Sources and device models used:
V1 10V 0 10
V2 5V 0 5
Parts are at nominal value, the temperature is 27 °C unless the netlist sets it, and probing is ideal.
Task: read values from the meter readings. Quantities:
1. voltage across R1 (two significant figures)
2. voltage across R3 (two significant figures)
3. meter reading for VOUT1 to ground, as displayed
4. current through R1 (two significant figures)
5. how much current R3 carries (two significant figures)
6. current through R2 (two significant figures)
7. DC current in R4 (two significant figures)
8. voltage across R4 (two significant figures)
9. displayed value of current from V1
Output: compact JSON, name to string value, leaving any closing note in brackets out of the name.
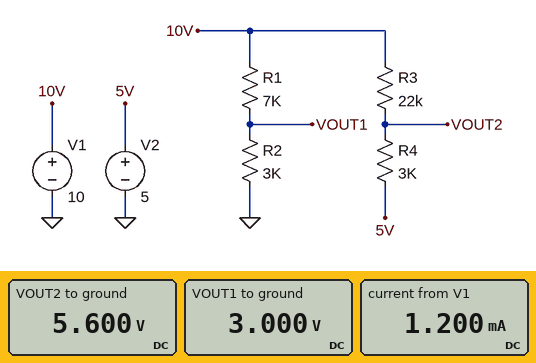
{"voltage across R1": "7.0 V", "voltage across R3": "4.4 V", "meter reading for VOUT1 to ground, as displayed": "3.000 V", "current through R1": "1.0 mA", "how much current R3 carries": "200 µA", "current through R2": "1.0 mA", "DC current in R4": "200 µA", "voltage across R4": "600 mV", "displayed value of current from V1": "1.200 mA"}
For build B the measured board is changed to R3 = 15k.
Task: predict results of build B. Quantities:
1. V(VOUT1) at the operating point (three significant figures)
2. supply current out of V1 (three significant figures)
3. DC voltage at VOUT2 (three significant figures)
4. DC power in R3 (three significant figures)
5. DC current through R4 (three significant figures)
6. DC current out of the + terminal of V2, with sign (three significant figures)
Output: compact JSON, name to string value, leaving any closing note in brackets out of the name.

{"V(VOUT1) at the operating point": "3.00 V", "supply current out of V1": "1.28 mA", "DC voltage at VOUT2": "5.83 V", "DC power in R3": "1.16 mW", "DC current through R4": "278 µA", "DC current out of the + terminal of V2, with sign": "-278 µA"}
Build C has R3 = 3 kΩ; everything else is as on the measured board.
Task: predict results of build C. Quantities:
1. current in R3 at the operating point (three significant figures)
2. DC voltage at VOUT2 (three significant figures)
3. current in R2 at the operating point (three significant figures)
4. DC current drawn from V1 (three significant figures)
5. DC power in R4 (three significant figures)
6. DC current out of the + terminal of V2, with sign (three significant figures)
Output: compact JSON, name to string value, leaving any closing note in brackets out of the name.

{"current in R3 at the operating point": "833 µA", "DC voltage at VOUT2": "7.50 V", "current in R2 at the operating point": "1.00 mA", "DC current drawn from V1": "1.83 mA", "DC power in R4": "2.08 mW", "DC current out of the + terminal of V2, with sign": "-833 µA"}
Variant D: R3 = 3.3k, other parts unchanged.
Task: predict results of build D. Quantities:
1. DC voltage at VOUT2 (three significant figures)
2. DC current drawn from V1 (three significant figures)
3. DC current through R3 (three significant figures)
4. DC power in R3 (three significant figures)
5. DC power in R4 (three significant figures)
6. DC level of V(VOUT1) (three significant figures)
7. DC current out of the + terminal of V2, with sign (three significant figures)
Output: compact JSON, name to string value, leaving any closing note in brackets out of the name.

{"DC voltage at VOUT2": "7.38 V", "DC current drawn from V1": "1.79 mA", "DC current through R3": "794 µA", "DC power in R3": "2.08 mW", "DC power in R4": "1.89 mW", "DC level of V(VOUT1)": "3.00 V", "DC current out of the + terminal of V2, with sign": "-794 µA"}
